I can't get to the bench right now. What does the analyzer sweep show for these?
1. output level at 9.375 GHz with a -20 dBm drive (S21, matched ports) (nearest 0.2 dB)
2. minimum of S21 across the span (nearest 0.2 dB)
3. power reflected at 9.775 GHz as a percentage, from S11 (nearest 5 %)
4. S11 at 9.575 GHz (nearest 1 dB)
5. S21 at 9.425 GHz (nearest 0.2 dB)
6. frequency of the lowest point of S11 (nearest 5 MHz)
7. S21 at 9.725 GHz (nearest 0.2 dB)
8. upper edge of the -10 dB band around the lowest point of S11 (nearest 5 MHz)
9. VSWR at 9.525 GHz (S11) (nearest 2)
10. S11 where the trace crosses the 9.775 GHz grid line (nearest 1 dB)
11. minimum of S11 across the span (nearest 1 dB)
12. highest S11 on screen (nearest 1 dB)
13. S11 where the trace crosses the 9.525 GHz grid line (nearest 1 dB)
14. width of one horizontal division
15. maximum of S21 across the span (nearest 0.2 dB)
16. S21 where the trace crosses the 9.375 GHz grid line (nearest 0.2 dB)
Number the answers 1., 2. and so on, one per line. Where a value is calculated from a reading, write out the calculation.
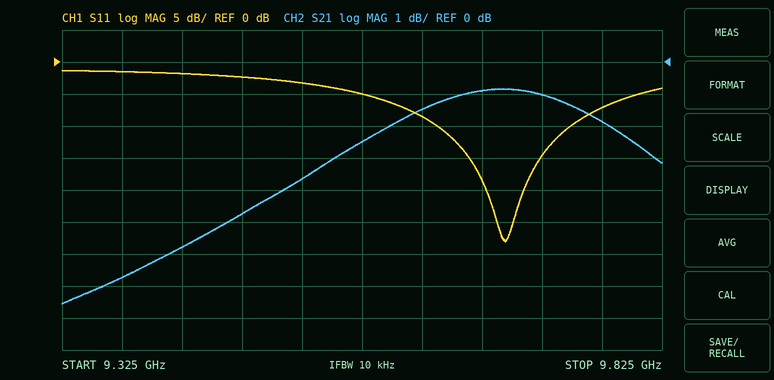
1. -20 dBm + (-6.8 dB) = -26.8 dBm
2. -7.6 dB
3. 10^(-7/10) ≈ 20 %
4. -5 dB
5. -5.8 dB
6. 9.695 GHz
7. -1.0 dB
8. 9.750 GHz
9. |Γ| = 10^(-3/20) = 0.7079; VSWR = (1 + 0.7079)/(1 − 0.7079) ≈ 6
10. -7 dB
11. -28 dB
12. -1 dB
13. -3 dB
14. 50 MHz
15. -0.8 dB
16. -6.8 dB
